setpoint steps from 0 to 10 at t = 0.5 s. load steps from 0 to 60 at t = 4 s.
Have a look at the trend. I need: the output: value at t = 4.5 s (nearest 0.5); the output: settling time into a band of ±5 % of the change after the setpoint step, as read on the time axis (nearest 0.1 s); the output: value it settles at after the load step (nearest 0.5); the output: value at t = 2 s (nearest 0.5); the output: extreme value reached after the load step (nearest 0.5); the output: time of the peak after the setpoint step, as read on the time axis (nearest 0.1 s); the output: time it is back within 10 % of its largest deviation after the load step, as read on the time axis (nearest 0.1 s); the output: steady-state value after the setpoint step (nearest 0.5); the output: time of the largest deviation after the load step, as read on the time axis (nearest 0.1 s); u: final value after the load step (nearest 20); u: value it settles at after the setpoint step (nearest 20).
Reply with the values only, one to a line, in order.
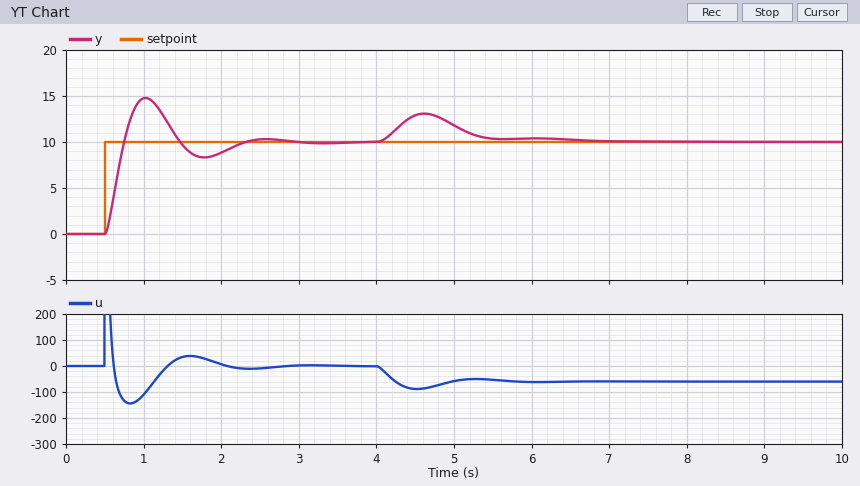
13.0
2.2 s
10.0
9.0
13.0
1.0 s
6.4 s
10.0
4.6 s
-60
0
